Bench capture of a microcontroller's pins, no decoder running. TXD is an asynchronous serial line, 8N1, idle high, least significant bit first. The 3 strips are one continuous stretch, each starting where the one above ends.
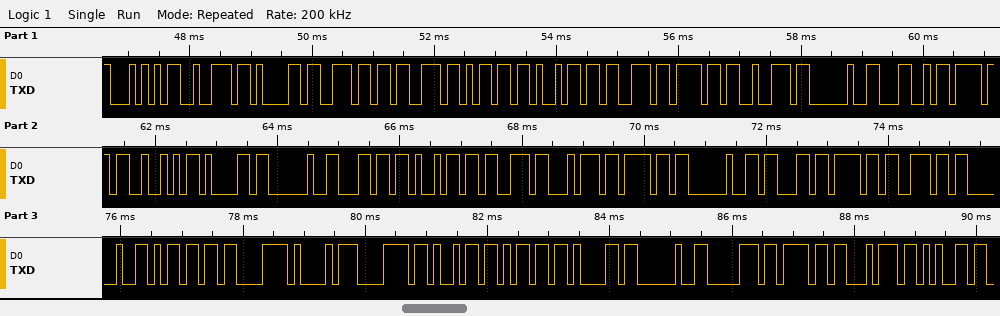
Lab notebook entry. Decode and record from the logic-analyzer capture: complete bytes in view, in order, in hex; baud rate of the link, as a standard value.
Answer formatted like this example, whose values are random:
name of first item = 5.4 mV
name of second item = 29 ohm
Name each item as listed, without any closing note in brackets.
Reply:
complete bytes in view, in order, in hex = 0x54 0x72 0x61 0x6E 0x73 0x6D 0x69 0x73 0x6F 0x72 0x20 0x4C 0x6F 0x52 0x61 0x20 0x6C 0x69 0x73 0x74 0x6F 0x20 0x63 0x6F 0x6E 0x20 0x6D 0xC3 0xA1 0x78 0x69 0x6D 0x61 0x20 0x70 0x6F 0x74 0x65
baud rate of the link, as a standard value = 9600 baud
